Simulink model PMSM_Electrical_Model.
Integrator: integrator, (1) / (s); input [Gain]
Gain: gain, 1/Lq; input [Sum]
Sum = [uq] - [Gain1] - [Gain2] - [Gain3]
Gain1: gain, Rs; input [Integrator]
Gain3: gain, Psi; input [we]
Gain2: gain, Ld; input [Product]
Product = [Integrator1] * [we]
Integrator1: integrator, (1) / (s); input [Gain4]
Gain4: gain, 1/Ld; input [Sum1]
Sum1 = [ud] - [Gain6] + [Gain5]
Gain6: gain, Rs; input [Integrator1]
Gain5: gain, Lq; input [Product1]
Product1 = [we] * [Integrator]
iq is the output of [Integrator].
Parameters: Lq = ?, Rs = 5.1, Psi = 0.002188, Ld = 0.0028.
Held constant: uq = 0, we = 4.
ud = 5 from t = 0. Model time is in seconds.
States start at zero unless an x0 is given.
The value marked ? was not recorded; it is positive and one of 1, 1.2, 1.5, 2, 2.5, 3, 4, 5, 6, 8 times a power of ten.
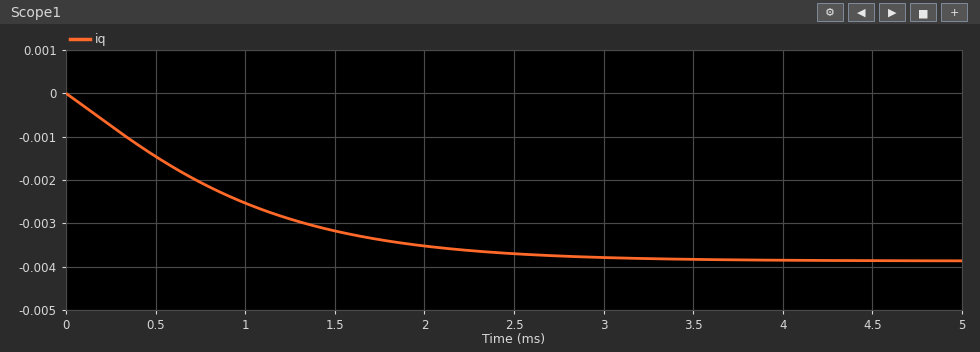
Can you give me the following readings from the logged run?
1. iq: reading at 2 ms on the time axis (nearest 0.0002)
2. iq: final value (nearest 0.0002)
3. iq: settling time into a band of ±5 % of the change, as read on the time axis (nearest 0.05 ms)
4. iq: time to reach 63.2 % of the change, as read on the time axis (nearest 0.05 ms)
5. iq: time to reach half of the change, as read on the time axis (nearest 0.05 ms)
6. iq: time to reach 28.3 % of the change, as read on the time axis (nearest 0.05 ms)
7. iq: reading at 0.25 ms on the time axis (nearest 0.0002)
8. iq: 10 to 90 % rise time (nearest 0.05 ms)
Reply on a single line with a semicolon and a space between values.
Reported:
-0.0036; -0.0038; 2.40 ms; 0.95 ms; 0.70 ms; 0.35 ms; -0.0008; 1.80 ms
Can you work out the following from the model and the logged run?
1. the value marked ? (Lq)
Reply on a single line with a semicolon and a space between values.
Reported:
0.003
